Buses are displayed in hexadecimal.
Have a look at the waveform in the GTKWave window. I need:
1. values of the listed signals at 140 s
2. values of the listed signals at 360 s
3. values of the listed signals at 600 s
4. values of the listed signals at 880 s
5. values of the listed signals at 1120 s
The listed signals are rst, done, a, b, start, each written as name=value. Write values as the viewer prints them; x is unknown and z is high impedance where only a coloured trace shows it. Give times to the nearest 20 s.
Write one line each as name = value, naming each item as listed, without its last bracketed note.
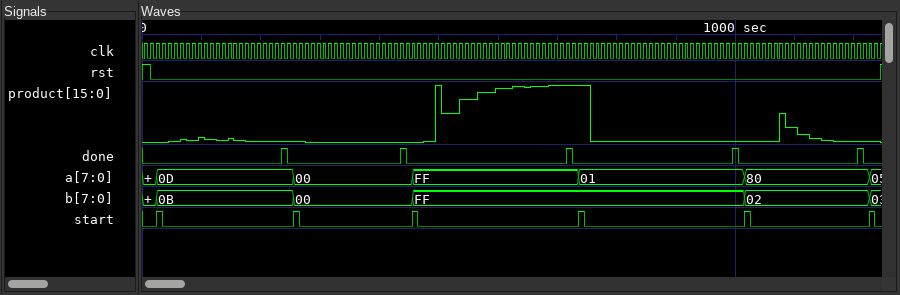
values of the listed signals at 140 s = rst=0, done=0, a=0D, b=0B, start=0
values of the listed signals at 360 s = rst=0, done=0, a=00, b=00, start=0
values of the listed signals at 600 s = rst=0, done=0, a=FF, b=FF, start=0
values of the listed signals at 880 s = rst=0, done=0, a=01, b=FF, start=0
values of the listed signals at 1120 s = rst=0, done=0, a=80, b=02, start=0
